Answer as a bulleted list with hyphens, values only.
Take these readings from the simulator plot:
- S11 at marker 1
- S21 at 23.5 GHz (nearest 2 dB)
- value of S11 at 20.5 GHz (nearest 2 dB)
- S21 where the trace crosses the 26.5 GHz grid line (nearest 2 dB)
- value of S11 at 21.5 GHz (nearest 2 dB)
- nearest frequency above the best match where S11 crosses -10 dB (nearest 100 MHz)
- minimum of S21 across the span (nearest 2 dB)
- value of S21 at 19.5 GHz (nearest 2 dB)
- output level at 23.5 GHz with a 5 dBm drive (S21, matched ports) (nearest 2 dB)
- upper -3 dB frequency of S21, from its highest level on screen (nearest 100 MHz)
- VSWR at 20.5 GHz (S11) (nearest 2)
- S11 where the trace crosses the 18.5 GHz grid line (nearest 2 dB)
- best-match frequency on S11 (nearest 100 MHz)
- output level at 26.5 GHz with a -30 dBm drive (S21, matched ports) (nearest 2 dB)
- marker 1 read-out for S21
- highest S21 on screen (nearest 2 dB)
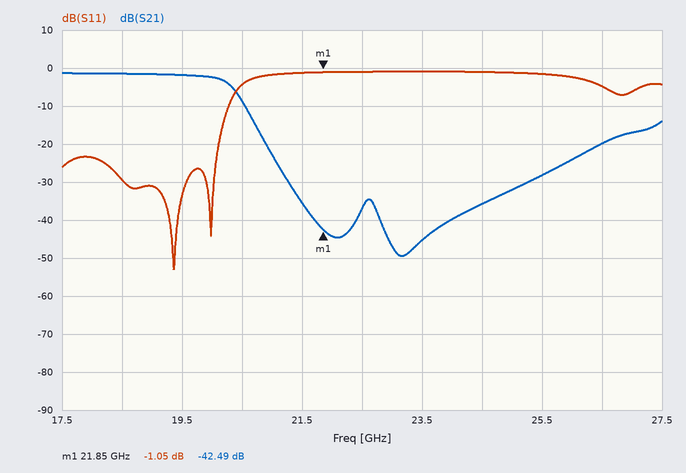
- -1.05 dB
- -46 dB
- -4 dB
- -20 dB
- -2 dB
- 20.3 GHz
- -50 dB
- -2 dB
- -40 dBm
- 20.3 GHz
- 4
- -30 dB
- 19.4 GHz
- -50 dBm
- -42.49 dB
- -2 dB
